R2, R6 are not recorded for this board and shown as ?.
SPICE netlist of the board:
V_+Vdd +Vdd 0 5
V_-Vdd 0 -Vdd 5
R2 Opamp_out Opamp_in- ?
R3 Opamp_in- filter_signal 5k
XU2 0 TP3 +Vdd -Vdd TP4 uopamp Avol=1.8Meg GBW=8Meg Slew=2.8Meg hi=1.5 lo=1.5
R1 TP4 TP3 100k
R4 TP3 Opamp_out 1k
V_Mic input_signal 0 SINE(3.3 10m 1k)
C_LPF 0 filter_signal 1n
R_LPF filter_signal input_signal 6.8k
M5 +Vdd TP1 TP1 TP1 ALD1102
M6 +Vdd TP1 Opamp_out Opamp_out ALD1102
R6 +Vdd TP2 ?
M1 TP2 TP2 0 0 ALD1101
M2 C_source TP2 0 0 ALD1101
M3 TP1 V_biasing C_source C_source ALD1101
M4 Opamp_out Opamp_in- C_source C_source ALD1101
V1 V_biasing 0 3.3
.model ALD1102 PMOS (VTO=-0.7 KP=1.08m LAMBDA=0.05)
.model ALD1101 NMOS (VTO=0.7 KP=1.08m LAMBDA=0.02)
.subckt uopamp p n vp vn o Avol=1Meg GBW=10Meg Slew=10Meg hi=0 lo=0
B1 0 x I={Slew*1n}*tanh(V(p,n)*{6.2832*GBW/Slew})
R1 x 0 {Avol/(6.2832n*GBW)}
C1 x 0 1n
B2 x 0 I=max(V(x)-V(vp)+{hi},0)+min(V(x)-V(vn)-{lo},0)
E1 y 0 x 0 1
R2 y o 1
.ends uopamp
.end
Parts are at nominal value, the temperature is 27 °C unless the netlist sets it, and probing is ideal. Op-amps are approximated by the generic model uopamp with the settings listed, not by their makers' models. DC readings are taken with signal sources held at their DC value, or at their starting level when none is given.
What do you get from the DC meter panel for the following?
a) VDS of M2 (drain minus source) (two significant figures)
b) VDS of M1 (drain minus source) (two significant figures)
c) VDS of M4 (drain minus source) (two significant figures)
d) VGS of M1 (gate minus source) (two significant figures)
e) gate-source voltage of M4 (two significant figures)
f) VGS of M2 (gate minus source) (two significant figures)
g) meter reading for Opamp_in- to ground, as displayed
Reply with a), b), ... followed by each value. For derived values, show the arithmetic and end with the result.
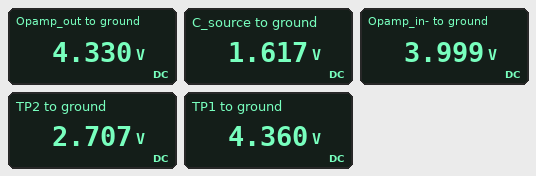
a) 1.617 V = 1.6 V
b) 2.707 V = 2.7 V
c) 4.33 V - 1.617 V = 2.7 V
d) 2.707 V = 2.7 V
e) 3.999 V - 1.617 V = 2.4 V
f) 2.707 V = 2.7 V
g) 3.999 V
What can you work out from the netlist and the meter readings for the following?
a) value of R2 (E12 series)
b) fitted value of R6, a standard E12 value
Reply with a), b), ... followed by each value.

a) 5.6 kΩ
b) 1 kΩ
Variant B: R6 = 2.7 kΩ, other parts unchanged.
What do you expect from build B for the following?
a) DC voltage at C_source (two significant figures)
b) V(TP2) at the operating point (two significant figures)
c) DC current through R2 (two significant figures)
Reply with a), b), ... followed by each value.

a) 2.0 V
b) 2.1 V
c) 60 µA
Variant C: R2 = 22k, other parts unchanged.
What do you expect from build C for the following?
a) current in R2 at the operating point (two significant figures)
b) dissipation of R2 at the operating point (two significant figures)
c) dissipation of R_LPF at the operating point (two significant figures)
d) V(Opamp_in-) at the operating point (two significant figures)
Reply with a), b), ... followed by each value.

a) 31 µA
b) 21 µW
c) 6.4 µW
d) 3.7 V
